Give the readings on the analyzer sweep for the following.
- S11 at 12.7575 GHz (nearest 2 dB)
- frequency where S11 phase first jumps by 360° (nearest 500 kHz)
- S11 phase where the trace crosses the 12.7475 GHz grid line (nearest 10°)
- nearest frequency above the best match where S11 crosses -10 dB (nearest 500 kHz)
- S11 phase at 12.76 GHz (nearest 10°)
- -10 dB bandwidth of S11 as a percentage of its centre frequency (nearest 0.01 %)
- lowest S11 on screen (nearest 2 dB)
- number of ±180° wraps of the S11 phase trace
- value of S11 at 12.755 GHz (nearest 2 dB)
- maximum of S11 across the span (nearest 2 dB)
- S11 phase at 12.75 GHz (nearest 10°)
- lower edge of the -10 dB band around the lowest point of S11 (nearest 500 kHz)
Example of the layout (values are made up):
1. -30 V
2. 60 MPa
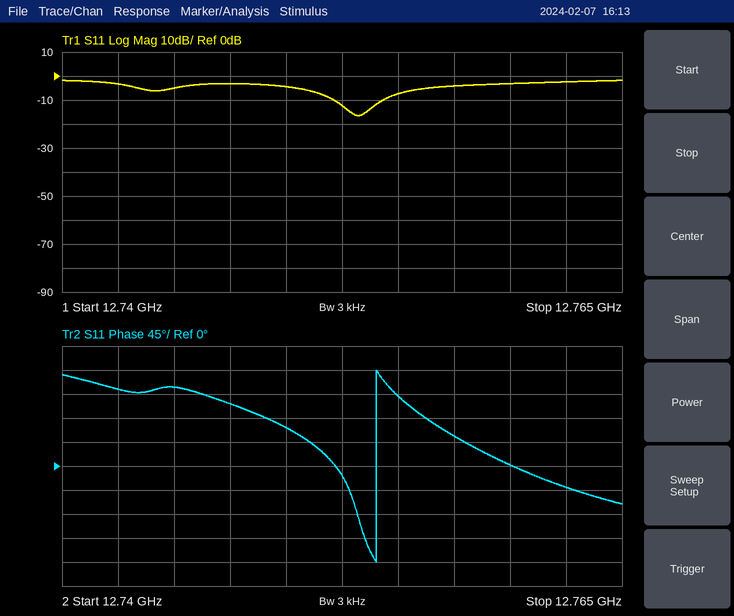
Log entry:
1. -4 dB
2. 12.7540 GHz
3. 120°
4. 12.7545 GHz
5. 0°
6. 0.02 %
7. -16 dB
8. 1
9. -8 dB
10. -2 dB
11. 70°
12. 12.7520 GHz
